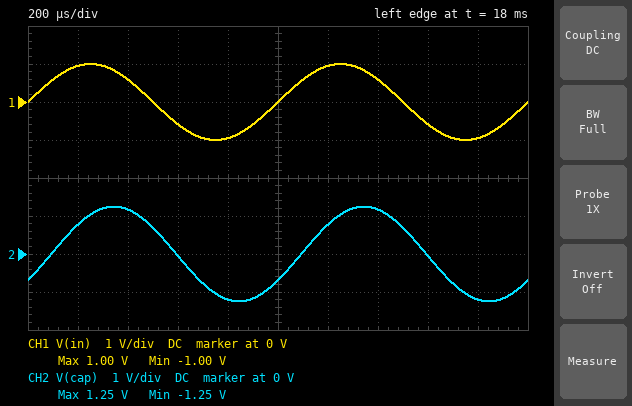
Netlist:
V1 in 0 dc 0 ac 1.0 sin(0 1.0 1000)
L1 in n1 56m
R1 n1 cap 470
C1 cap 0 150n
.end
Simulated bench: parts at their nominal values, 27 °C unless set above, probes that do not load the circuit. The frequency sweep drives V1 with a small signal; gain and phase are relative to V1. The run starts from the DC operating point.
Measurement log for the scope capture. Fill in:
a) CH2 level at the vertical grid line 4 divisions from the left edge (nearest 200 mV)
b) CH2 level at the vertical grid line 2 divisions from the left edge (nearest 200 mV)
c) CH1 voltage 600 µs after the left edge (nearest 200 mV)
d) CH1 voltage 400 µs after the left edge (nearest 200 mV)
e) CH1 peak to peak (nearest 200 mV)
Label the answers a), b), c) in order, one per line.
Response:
a) -1.2 V
b) 1.2 V
c) -600 mV
d) 600 mV
e) 2.0 V
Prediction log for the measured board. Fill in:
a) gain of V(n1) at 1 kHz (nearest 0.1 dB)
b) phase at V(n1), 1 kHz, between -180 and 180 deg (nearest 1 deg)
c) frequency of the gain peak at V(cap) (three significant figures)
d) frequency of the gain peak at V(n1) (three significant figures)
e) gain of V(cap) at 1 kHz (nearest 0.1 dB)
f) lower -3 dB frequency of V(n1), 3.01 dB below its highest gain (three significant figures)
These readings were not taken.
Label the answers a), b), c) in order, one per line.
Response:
a) 2.7 dB
b) -10 deg
c) 1.46 kHz
d) 1.56 kHz
e) 1.9 dB
f) 748 Hz
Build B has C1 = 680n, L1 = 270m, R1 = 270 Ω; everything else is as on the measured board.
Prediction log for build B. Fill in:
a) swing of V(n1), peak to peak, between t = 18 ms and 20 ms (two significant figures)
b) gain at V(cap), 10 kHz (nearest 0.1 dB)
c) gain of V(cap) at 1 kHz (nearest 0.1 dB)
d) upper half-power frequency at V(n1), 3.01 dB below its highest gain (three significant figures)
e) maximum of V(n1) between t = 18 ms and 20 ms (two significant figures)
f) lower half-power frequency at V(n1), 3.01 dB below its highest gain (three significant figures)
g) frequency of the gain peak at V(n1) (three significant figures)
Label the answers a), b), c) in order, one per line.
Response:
a) 480 mV
b) -57.2 dB
c) -16.1 dB
d) 432 Hz
e) 240 mV
f) 267 Hz
g) 357 Hz
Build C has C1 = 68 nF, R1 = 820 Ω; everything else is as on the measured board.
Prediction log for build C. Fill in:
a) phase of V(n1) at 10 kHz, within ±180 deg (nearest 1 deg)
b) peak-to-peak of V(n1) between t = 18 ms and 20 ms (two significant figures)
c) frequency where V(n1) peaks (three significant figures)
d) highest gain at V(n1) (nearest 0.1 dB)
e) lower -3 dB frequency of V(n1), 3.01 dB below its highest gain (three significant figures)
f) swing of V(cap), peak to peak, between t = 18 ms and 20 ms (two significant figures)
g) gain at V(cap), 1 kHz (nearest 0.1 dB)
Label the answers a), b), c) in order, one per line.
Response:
a) -92 deg
b) 2.3 V
c) 2.25 kHz
d) 3.8 dB
e) 782 Hz
f) 2.2 V
g) 0.7 dB
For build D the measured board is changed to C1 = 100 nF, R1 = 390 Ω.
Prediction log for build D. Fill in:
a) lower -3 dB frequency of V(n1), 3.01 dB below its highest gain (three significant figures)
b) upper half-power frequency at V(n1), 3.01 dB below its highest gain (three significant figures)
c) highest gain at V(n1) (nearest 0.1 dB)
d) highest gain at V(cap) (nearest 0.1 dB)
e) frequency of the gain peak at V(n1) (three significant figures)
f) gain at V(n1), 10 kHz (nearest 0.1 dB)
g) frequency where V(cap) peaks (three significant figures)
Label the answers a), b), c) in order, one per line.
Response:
a) 1.37 kHz
b) 2.54 kHz
c) 6.9 dB
d) 6.0 dB
e) 2.01 kHz
f) -18.1 dB
g) 1.98 kHz
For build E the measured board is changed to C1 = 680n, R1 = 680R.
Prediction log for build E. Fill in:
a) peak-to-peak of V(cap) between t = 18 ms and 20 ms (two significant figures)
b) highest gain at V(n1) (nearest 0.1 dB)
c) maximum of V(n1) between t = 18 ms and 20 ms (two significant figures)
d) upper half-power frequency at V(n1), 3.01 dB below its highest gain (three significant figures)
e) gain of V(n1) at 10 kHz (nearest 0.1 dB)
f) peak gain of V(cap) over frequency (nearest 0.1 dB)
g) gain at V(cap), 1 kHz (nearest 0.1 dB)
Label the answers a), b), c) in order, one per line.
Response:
a) 680 mV
b) 1.0 dB
c) 1.0 V
d) 1.91 kHz
e) -14.4 dB
f) 0 dB
g) -9.4 dB
